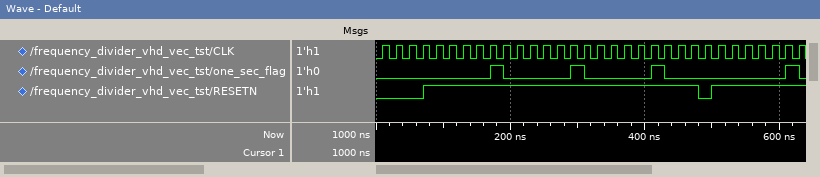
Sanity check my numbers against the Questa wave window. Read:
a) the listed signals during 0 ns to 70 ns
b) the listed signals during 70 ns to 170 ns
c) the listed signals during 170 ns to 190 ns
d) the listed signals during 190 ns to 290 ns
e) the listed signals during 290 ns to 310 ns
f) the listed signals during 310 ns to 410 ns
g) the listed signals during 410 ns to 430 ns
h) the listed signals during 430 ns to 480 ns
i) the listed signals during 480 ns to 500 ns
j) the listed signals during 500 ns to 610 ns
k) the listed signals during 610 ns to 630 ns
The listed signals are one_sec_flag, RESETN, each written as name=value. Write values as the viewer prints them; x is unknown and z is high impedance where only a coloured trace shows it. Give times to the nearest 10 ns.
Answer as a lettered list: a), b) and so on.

a) one_sec_flag=0, RESETN=0
b) one_sec_flag=0, RESETN=1
c) one_sec_flag=1, RESETN=1
d) one_sec_flag=0, RESETN=1
e) one_sec_flag=1, RESETN=1
f) one_sec_flag=0, RESETN=1
g) one_sec_flag=1, RESETN=1
h) one_sec_flag=0, RESETN=1
i) one_sec_flag=0, RESETN=0
j) one_sec_flag=0, RESETN=1
k) one_sec_flag=1, RESETN=1
